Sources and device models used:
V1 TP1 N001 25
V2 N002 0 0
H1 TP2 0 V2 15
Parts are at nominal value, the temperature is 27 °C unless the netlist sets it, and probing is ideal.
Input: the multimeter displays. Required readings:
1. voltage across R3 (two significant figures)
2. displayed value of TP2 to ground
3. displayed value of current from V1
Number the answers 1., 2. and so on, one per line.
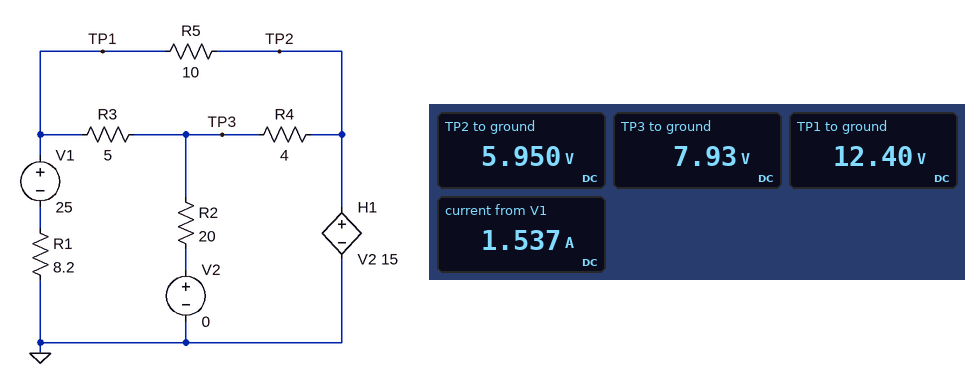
1. 4.5 V
2. 5.950 V
3. 1.537 A
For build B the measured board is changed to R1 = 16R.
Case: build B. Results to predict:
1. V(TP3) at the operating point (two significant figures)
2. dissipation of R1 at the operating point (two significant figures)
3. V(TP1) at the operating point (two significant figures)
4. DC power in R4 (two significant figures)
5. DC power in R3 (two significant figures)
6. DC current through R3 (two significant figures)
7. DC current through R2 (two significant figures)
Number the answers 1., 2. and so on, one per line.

1. 5.4 V
2. 17 W
3. 8.4 V
4. 450 mW
5. 1.8 W
6. 600 mA
7. 270 mA
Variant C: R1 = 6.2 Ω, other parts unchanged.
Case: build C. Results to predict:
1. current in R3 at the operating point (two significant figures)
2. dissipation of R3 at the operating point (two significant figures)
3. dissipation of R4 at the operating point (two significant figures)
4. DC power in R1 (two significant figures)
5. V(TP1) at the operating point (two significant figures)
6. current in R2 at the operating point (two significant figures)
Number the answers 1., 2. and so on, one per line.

1. 1.0 A
2. 5.2 W
3. 1.3 W
4. 19 W
5. 14 V
6. 450 mA
